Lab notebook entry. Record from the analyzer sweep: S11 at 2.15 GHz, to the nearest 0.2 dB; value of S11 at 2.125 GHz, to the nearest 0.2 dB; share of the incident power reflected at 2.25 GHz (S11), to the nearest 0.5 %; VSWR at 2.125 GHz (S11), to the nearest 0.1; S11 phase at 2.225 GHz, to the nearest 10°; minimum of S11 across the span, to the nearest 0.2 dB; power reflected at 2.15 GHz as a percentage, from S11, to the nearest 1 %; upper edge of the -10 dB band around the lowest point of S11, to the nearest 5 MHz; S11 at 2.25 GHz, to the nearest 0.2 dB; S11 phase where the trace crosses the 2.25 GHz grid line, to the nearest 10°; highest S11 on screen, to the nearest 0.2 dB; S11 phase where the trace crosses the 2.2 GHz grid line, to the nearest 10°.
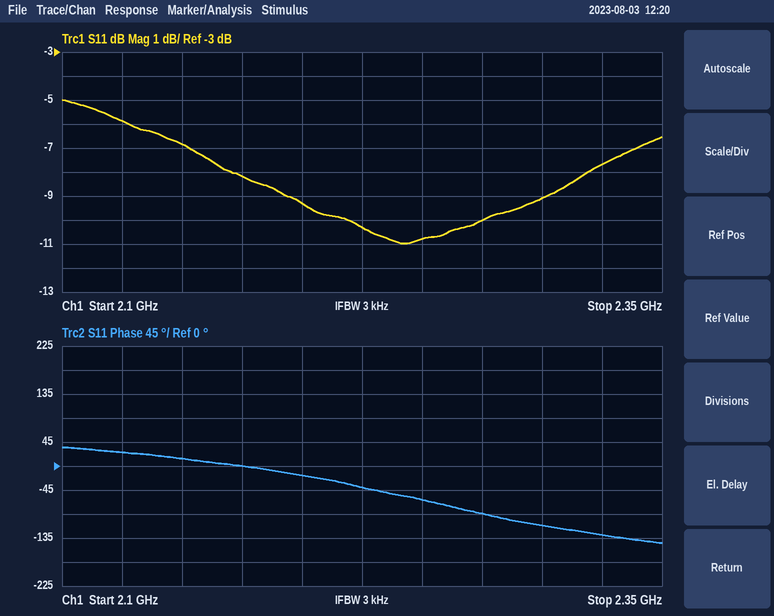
-6.8 dB
-5.8 dB
8.5 %
3.1
-40°
-11.0 dB
21 %
2.275 GHz
-10.8 dB
-60°
-5.0 dB
-20°
